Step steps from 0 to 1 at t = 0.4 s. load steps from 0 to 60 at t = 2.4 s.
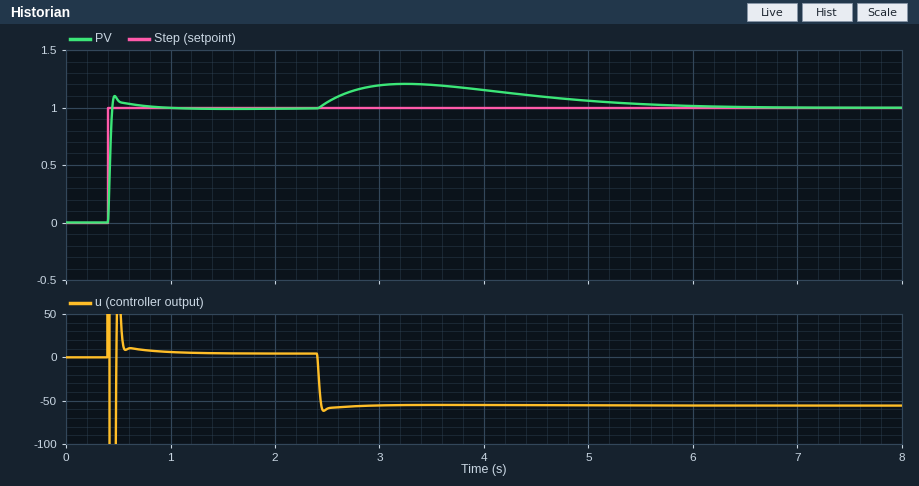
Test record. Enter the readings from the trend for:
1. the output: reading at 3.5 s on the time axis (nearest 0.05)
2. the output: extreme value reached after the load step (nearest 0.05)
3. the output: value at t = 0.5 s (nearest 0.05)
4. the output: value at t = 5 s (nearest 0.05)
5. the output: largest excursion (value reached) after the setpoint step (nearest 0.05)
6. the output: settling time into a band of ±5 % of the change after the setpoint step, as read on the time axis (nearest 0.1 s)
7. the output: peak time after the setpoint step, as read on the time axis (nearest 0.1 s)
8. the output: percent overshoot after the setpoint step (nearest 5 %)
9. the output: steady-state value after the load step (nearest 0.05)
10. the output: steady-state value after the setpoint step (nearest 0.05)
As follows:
1.20
1.20
1.05
1.05
1.10
0.5 s
0.5 s
10 %
1.00
1.00
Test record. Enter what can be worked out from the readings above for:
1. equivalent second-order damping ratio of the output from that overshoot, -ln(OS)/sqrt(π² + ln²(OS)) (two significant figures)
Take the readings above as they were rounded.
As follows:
0.59
